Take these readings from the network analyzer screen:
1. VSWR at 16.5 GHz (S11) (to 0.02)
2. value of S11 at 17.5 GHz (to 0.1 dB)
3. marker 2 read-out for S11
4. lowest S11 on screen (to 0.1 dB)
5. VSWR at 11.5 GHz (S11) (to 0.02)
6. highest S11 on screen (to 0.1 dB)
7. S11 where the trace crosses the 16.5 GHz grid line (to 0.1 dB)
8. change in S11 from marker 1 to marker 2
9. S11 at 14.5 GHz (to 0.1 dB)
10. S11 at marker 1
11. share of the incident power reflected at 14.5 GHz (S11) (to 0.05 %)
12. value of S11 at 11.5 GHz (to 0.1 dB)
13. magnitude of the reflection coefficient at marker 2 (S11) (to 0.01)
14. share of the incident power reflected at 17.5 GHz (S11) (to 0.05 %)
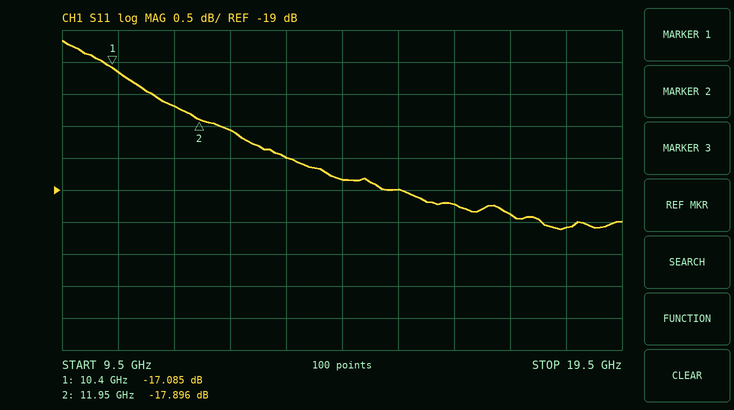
1.24
-19.4 dB
-17.896 dB
-19.6 dB
1.30
-16.7 dB
-19.2 dB
-0.811 dB
-18.8 dB
-17.085 dB
1.30 %
-17.7 dB
0.13
1.15 %
